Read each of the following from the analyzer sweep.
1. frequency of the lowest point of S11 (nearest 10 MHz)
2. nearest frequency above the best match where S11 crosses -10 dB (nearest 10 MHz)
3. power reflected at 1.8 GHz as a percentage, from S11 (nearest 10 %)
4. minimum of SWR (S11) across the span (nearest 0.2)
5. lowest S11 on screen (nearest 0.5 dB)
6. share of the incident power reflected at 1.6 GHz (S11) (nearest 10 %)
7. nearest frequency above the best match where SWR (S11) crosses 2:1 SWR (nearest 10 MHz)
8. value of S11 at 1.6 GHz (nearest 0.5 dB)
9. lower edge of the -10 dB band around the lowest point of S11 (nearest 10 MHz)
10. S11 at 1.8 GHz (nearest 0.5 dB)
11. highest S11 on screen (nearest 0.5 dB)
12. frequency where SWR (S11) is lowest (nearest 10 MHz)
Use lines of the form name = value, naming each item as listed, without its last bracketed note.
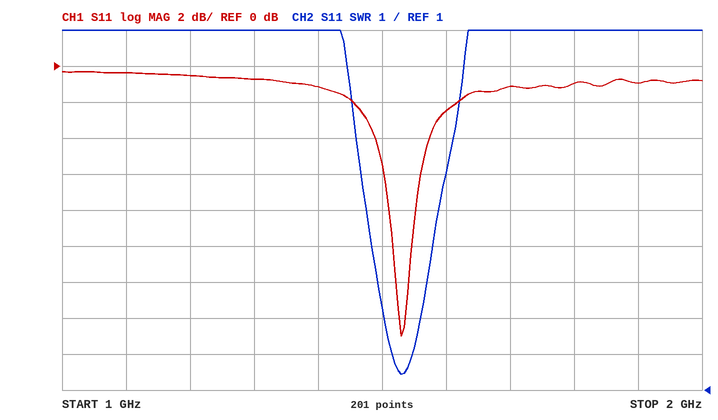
frequency of the lowest point of S11 = 1.53 GHz
nearest frequency above the best match where S11 crosses -10 dB = 1.55 GHz
power reflected at 1.8 GHz as a percentage, from S11 = 80 %
minimum of SWR (S11) across the span = 1.4
lowest S11 on screen = -15.0 dB
share of the incident power reflected at 1.6 GHz (S11) = 60 %
nearest frequency above the best match where SWR (S11) crosses 2:1 SWR = 1.55 GHz
value of S11 at 1.6 GHz = -2.5 dB
lower edge of the -10 dB band around the lowest point of S11 = 1.52 GHz
S11 at 1.8 GHz = -1.0 dB
highest S11 on screen = -0.5 dB
frequency where SWR (S11) is lowest = 1.53 GHz
